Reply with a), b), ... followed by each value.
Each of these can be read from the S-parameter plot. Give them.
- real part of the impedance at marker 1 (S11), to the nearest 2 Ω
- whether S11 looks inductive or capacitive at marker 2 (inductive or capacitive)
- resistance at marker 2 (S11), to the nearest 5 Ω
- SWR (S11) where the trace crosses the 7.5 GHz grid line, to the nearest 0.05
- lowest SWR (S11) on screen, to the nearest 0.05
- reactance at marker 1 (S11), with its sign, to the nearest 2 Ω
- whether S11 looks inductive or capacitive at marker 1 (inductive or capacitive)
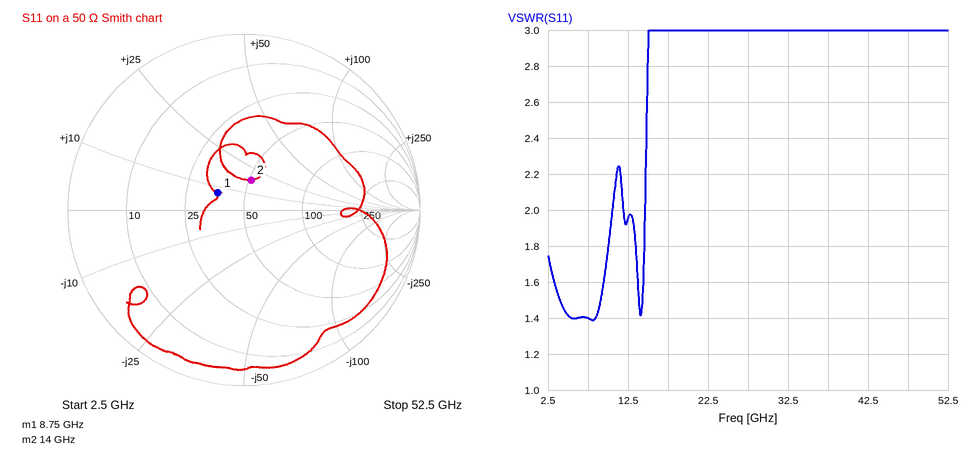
a) 36 Ω
b) inductive
c) 50 Ω
d) 1.40
e) 1.40
f) +8 Ω
g) inductive
